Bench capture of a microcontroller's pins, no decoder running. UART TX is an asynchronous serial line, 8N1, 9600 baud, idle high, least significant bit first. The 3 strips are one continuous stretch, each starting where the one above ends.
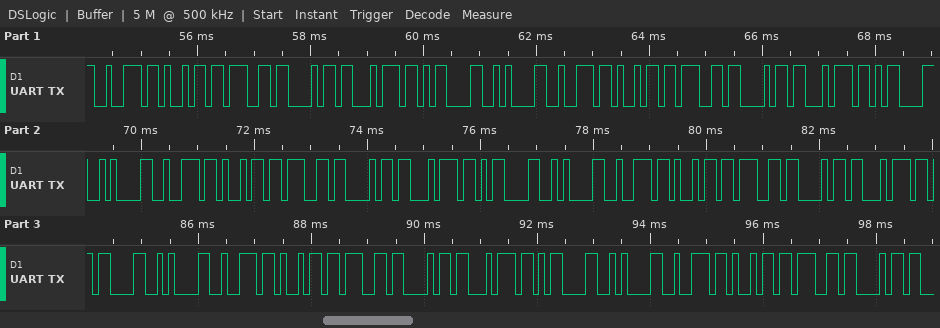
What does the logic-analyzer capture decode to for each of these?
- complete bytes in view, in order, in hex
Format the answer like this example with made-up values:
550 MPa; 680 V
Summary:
72 69 67 68 74 0D 0A 72 69 67 68 74 0D 0A 72 69 67 68 74 0D 0A 72 69 67 68 74 0D 0A 72 69 67 68 74 0D 0A 72 69 67 68
